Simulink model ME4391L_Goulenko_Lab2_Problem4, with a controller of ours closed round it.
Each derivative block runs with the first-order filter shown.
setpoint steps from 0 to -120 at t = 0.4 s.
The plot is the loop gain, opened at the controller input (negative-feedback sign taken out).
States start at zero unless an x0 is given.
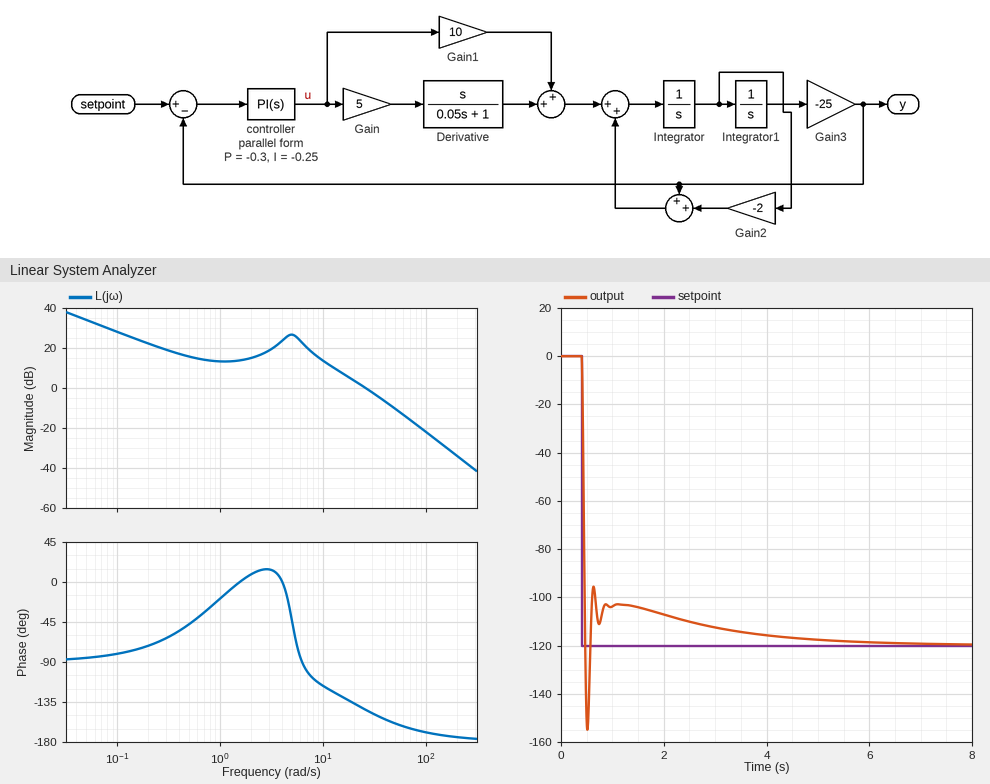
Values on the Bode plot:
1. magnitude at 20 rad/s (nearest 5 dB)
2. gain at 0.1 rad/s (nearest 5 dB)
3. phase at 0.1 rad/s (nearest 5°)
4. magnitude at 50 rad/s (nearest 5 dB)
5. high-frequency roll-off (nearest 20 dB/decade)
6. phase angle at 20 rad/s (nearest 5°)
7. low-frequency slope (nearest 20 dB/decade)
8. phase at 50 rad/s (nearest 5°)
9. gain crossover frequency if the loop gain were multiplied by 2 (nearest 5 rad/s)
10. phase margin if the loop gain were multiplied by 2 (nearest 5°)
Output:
5 dB
30 dB
-80°
-10 dB
-40 dB/decade
-135°
-20 dB/decade
-160°
40 rad/s
25°
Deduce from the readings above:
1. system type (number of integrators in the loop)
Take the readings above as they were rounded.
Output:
1
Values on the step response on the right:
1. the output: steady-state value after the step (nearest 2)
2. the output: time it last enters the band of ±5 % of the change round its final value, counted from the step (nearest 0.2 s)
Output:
-120
3.0 s
